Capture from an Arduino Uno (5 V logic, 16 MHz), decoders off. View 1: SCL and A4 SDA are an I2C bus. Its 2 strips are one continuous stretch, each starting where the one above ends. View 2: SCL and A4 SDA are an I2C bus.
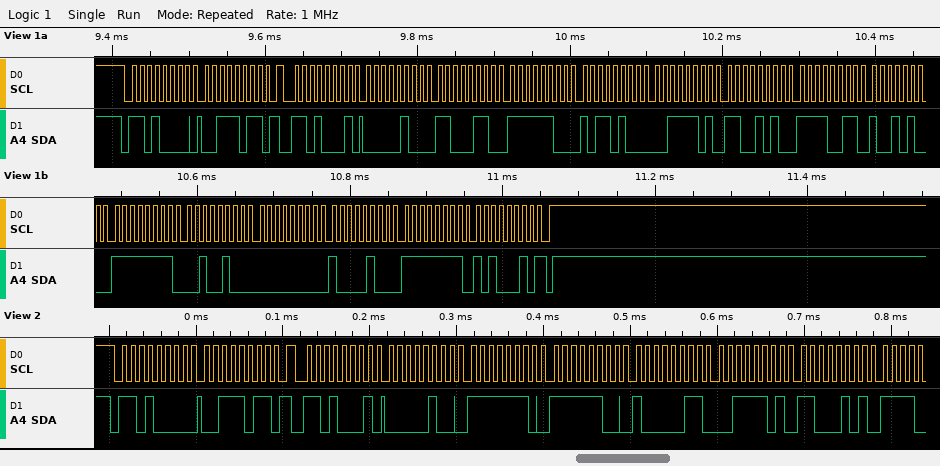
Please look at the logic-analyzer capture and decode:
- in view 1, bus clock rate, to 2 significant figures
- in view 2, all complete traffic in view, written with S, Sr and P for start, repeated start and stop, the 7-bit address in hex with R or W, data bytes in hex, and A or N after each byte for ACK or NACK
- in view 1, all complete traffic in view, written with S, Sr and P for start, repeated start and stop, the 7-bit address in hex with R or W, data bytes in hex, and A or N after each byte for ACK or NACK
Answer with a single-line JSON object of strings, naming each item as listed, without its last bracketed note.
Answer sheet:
{"in view 1, bus clock rate, to 2 significant figures": "100 kHz", "in view 2, all complete traffic in view, written with S, Sr and P for start, repeated start and stop, the 7-bit address in hex with R or W, data bytes in hex, and A or N after each byte for ACK or NACK": "S 68W A 3B A Sr 68R A 04 A FE A FC A 83 A 3D A C5 A", "in view 1, all complete traffic in view, written with S, Sr and P for start, repeated start and stop, the 7-bit address in hex with R or W, data bytes in hex, and A or N after each byte for ACK or NACK": "S 68W A 3B A Sr 68R A 04 A C6 A FC A B4 A 3D A CA A F3 A 94 A FF A 24 A 00 A 84 A FF A A2 N P"}
